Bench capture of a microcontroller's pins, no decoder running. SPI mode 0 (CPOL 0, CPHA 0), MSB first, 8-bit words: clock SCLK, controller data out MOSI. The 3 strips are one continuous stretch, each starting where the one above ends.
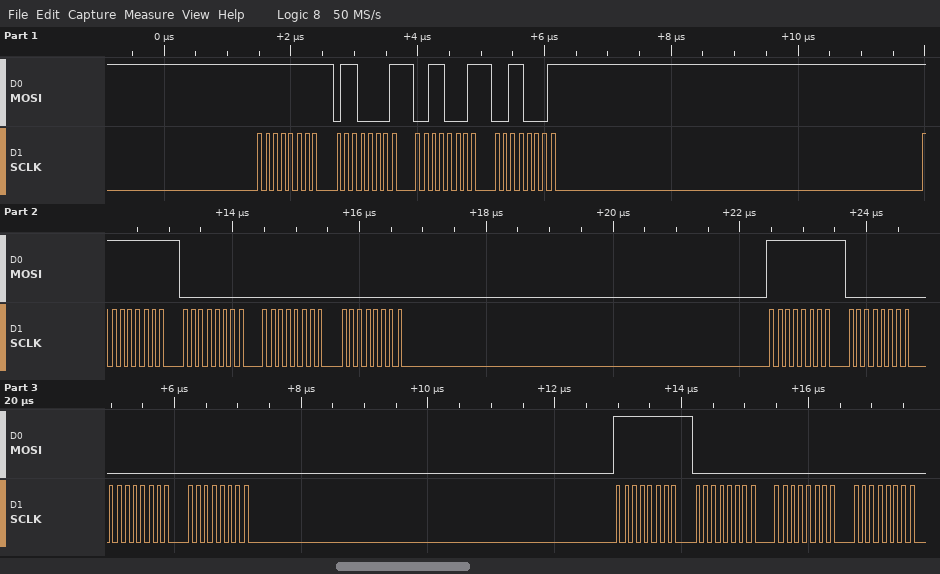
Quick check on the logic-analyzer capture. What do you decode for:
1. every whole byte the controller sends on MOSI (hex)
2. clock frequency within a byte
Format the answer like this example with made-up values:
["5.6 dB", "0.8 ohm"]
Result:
["FF 61 31 31 FF 00 00 00 FF 00 00 00 FF 00 00 00", "8 MHz"]
